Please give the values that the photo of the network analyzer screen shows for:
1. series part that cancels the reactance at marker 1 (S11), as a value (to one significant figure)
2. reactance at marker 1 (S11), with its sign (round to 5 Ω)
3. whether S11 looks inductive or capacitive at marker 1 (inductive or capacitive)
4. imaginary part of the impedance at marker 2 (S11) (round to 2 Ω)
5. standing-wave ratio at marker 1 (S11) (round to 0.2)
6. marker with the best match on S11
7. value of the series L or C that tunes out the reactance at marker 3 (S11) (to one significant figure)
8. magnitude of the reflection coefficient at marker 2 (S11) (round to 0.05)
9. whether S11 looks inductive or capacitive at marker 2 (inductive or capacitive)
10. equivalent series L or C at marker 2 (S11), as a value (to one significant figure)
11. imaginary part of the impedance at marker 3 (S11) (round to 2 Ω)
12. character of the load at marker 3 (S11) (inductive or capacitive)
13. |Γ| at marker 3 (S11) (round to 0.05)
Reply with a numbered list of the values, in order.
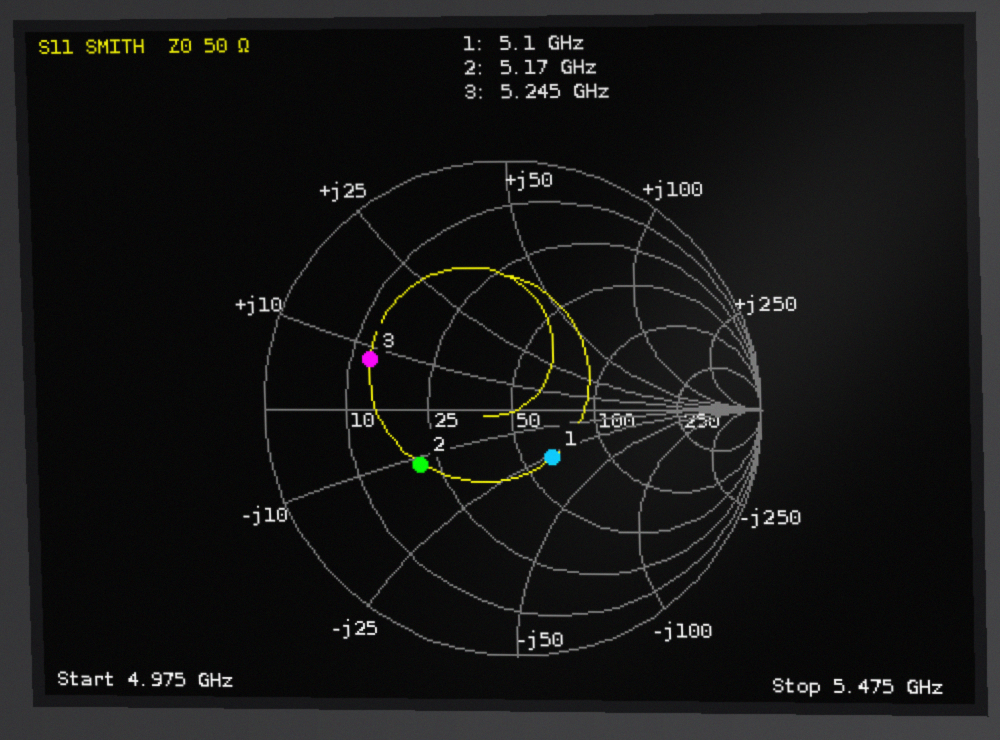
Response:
1. 800 pH
2. -25 Ω
3. capacitive
4. -12 Ω
5. 1.6
6. marker 1
7. 4 pF
8. 0.45
9. capacitive
10. 3 pF
11. +8 Ω
12. inductive
13. 0.60
